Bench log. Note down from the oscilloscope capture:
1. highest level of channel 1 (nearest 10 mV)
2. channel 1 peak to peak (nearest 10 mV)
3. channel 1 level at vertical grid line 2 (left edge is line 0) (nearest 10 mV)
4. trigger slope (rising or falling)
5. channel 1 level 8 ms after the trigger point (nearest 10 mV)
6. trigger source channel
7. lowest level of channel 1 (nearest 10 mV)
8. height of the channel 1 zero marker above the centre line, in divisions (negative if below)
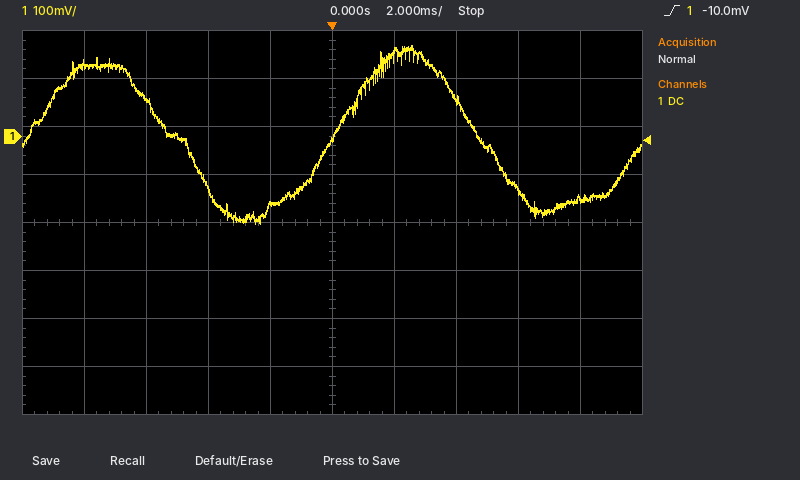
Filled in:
190 mV
370 mV
80 mV
rising
-130 mV
channel 1
-180 mV
+1.8 div
